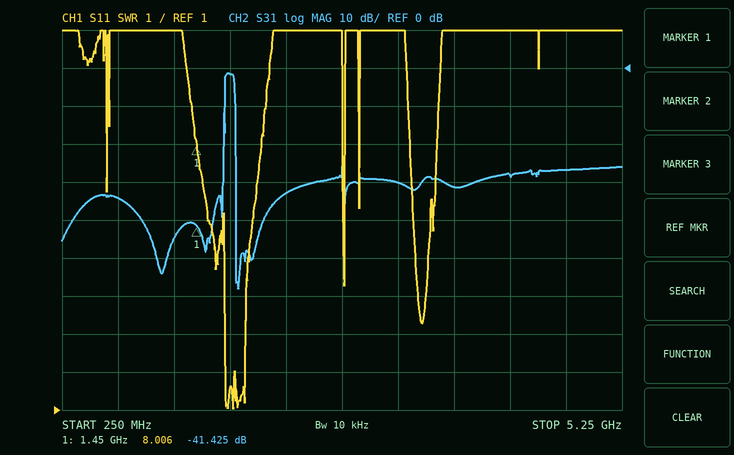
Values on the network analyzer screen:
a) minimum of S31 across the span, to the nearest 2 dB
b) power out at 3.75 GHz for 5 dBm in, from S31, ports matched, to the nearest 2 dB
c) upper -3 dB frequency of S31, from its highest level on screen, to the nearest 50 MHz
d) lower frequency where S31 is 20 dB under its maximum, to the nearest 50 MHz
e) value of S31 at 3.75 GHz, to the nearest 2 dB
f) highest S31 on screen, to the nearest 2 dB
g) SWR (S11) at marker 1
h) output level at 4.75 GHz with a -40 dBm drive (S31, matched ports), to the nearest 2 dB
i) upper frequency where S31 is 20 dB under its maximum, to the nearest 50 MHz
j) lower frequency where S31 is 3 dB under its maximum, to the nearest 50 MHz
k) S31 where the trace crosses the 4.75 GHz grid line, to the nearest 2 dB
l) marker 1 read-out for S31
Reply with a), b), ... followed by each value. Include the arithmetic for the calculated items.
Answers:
a) -58 dB
b) 5 dBm + (-32 dB) = -26 dBm
c) 1.80 GHz
d) 1.70 GHz
e) -32 dB
f) -2 dB
g) 8.006
h) -40 dBm + (-26 dB) = -66 dBm
i) 1.80 GHz
j) 1.70 GHz
k) -26 dB
l) -41.425 dB
